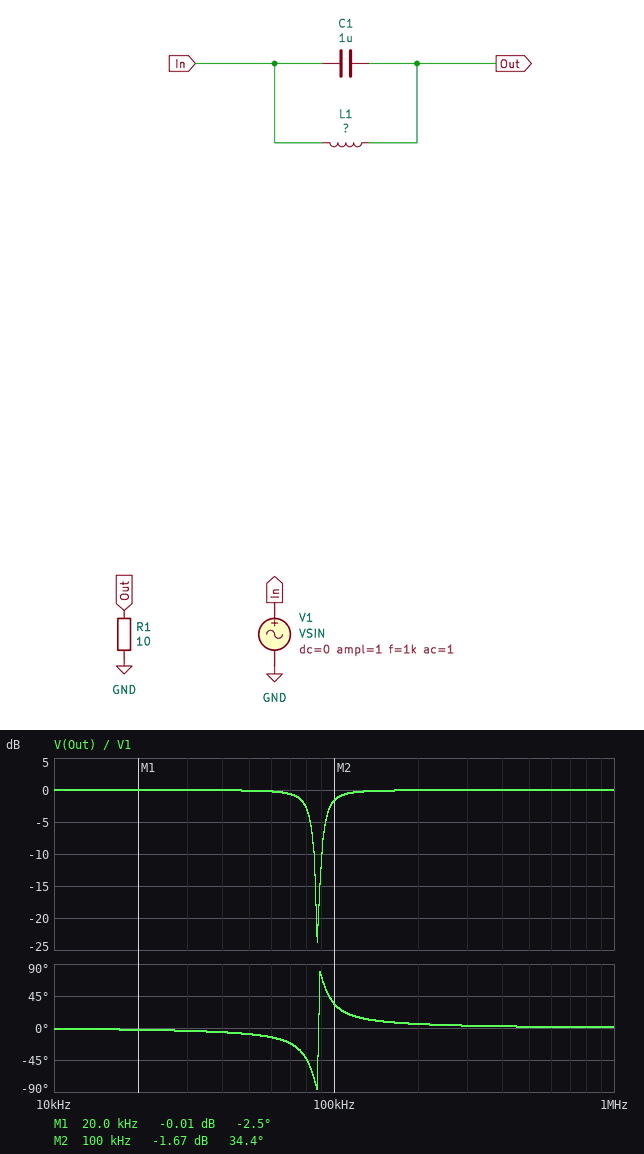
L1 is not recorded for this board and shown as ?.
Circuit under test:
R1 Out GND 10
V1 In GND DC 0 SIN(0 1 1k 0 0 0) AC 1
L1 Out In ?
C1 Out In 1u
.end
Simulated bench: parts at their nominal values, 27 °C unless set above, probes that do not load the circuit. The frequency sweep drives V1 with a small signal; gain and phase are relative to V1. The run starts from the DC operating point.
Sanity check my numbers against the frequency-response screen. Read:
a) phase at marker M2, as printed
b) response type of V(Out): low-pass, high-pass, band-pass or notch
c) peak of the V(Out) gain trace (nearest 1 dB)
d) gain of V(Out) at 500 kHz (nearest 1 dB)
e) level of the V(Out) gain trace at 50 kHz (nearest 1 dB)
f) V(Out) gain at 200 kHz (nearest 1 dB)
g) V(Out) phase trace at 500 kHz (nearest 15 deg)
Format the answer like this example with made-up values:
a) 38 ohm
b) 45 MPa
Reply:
a) 34.4 deg
b) notch
c) 0 dB
d) 0 dB
e) 0 dB
f) 0 dB
g) 0 deg
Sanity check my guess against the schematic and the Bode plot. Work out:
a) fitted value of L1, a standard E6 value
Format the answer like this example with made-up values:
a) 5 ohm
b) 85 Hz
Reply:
a) 3.3 µH
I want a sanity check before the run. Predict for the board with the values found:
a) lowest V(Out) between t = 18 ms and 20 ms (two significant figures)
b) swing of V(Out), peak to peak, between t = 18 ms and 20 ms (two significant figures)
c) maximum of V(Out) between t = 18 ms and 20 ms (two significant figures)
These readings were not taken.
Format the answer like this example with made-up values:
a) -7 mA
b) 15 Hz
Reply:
a) -1.0 V
b) 2.0 V
c) 1.0 V
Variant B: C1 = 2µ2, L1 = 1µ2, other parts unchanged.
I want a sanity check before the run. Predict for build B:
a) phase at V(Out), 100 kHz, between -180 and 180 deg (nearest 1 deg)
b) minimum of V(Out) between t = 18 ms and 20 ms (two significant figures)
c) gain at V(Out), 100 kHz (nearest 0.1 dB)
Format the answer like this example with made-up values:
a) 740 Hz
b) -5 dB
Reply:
a) 61 deg
b) -1.0 V
c) -6.2 dB
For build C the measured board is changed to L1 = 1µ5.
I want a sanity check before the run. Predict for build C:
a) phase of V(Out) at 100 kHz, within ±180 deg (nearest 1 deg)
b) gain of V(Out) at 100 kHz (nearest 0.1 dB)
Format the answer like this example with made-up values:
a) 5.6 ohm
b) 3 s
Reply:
a) -13 deg
b) -0.2 dB
